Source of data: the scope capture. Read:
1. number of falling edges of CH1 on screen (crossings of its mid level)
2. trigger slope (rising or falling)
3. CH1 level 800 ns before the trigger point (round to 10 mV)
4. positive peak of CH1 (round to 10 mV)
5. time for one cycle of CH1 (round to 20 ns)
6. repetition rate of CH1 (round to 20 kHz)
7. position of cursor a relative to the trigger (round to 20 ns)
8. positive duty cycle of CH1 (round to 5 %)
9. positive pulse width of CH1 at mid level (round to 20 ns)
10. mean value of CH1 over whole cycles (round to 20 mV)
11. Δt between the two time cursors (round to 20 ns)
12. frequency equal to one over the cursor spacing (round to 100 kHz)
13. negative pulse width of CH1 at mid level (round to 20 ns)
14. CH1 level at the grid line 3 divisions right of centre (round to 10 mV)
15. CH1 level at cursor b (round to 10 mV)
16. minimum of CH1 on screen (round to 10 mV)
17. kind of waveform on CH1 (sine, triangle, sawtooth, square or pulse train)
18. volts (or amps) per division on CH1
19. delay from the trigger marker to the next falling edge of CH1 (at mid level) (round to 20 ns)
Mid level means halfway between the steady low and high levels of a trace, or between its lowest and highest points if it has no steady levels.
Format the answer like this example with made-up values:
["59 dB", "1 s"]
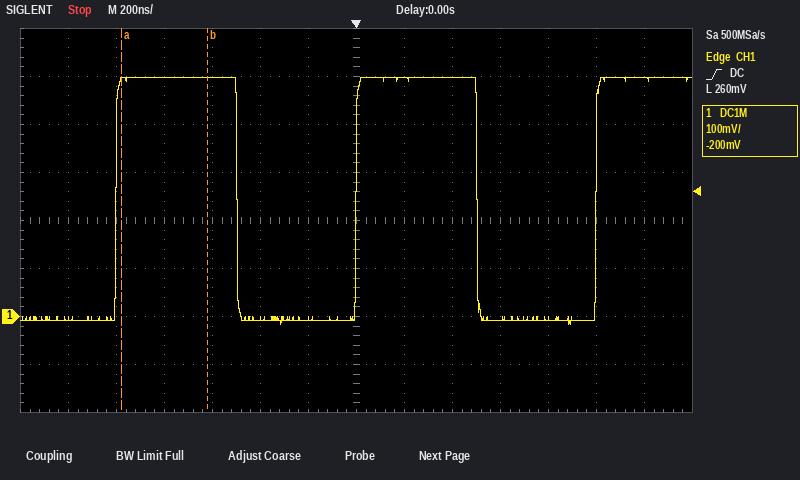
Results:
["2", "rising", "500 mV", "500 mV", "1.00 µs", "1.00 MHz", "-980 ns", "50 %", "500 ns", "240 mV", "360 ns", "2.8 MHz", "500 ns", "-10 mV", "500 mV", "-20 mV", "square", "100 mV", "500 ns"]
